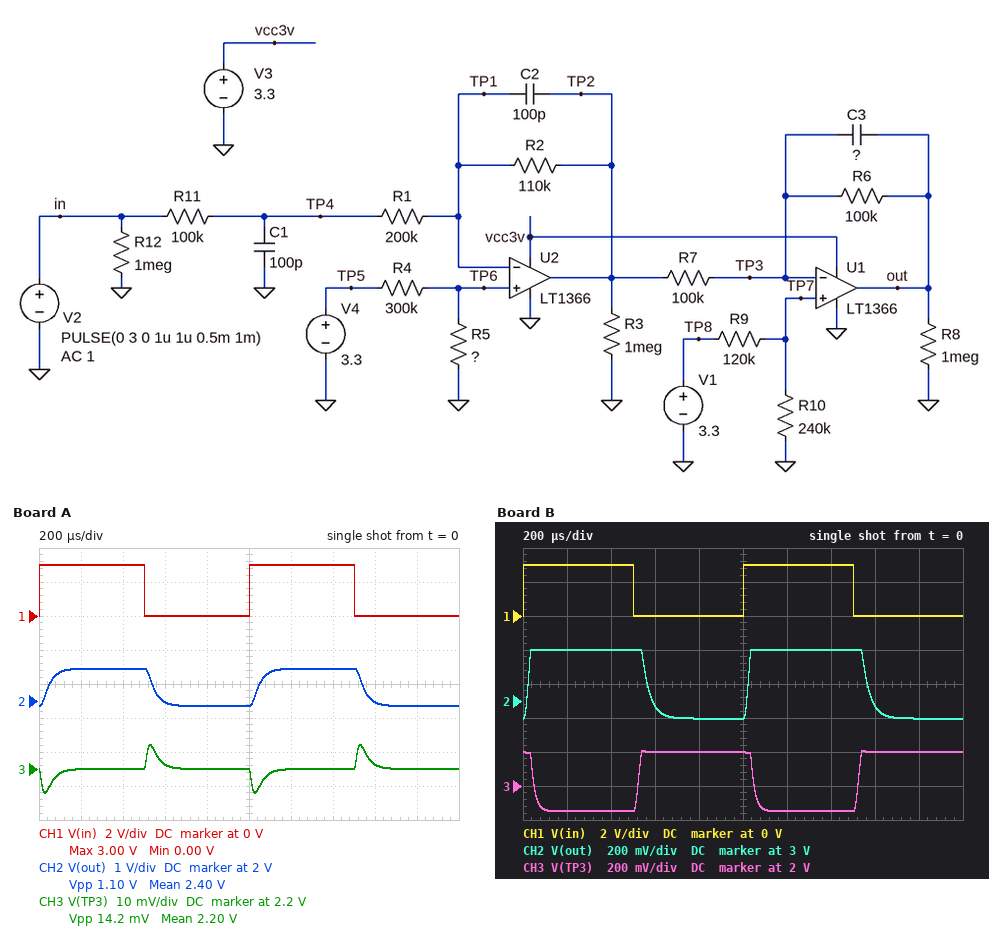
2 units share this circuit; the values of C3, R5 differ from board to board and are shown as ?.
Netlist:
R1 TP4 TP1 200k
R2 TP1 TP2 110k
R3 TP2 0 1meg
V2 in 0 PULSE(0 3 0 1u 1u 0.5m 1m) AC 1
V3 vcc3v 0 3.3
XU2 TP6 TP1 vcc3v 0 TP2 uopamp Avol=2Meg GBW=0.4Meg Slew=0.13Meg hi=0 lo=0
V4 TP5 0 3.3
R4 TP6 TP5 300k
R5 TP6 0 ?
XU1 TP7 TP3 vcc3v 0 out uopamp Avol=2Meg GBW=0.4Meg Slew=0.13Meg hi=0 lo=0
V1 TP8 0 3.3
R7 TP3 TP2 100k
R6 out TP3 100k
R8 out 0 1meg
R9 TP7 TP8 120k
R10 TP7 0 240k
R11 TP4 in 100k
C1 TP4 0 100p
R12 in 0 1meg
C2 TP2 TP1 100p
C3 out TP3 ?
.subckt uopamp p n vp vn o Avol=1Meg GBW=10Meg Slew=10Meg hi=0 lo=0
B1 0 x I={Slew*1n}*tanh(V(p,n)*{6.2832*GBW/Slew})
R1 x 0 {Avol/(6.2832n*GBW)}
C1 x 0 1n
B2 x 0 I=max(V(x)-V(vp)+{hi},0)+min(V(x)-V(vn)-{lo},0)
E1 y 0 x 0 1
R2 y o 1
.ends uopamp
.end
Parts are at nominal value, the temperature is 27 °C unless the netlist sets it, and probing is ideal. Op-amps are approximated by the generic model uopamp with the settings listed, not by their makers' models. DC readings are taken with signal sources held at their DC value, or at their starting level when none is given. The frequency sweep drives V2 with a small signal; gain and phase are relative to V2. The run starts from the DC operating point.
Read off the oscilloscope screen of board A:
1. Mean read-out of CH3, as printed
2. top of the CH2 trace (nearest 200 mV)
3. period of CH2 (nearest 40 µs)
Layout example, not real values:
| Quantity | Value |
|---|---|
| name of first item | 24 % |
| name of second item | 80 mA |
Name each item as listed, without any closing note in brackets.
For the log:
| Quantity | Value |
|---|---|
| Mean read-out of CH3, as printed | 2.20 V |
| top of the CH2 trace | 3.0 V |
| period of CH2 | 1.00 ms |
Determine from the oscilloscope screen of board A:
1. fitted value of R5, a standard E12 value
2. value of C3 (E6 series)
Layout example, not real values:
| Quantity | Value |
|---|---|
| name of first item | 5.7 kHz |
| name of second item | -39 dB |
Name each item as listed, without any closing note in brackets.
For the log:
| Quantity | Value |
|---|---|
| fitted value of R5, a standard E12 value | 390 kΩ |
| value of C3 | 330 pF |
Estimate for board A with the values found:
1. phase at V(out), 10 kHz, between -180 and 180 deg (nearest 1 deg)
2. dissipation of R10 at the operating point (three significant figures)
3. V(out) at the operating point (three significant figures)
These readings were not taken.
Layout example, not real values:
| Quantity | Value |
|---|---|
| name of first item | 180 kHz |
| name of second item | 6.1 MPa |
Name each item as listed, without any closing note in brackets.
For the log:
| Quantity | Value |
|---|---|
| phase at V(out), 10 kHz, between -180 and 180 deg | -125 deg |
| dissipation of R10 at the operating point | 20.2 µW |
| V(out) at the operating point | 1.85 V |
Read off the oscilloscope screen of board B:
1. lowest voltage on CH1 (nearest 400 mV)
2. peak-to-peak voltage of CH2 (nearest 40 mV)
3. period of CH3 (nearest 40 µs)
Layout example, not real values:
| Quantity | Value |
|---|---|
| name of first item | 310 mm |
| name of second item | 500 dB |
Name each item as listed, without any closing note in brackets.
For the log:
| Quantity | Value |
|---|---|
| lowest voltage on CH1 | 0 V |
| peak-to-peak voltage of CH2 | 400 mV |
| period of CH3 | 1.00 ms |
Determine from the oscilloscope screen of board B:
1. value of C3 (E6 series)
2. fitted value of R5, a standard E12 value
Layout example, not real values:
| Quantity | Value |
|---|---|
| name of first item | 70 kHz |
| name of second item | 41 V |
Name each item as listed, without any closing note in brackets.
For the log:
| Quantity | Value |
|---|---|
| value of C3 | 330 pF |
| fitted value of R5, a standard E12 value | 150 kΩ |
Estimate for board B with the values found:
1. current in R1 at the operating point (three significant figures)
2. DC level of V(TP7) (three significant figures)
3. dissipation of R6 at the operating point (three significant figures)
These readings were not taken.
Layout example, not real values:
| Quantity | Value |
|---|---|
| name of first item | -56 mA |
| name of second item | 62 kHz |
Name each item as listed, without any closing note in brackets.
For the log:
| Quantity | Value |
|---|---|
| current in R1 at the operating point | 3.67 µA |
| DC level of V(TP7) | 2.20 V |
| dissipation of R6 at the operating point | 4.85 µW |
